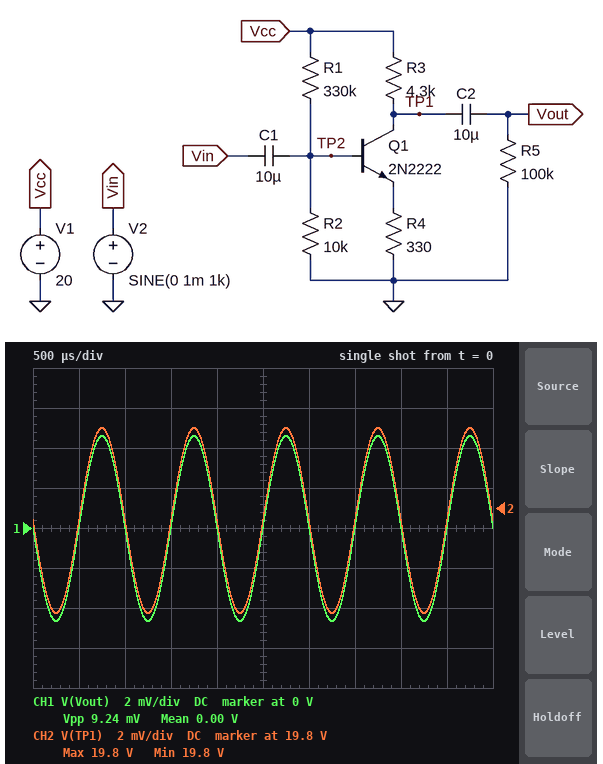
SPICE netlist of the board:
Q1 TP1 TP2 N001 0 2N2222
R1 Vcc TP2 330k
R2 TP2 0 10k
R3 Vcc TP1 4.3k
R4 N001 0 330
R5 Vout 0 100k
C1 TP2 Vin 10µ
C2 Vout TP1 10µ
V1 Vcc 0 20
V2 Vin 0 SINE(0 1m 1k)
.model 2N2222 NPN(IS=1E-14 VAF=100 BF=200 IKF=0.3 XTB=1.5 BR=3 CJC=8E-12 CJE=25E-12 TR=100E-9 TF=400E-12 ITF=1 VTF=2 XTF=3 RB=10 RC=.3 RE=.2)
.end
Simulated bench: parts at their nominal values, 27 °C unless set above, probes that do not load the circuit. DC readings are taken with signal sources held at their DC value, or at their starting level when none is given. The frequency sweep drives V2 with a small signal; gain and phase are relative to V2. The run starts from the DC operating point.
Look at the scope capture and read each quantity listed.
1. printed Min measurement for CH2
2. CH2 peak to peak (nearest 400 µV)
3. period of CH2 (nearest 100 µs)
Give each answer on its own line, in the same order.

19.8 V
9.2 mV
1.0 ms
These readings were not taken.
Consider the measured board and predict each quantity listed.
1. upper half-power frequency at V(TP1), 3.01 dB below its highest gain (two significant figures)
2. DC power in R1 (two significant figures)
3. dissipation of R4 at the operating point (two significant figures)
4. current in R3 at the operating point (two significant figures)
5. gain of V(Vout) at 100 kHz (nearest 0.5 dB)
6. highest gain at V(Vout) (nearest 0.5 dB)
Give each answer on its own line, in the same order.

13 MHz
1.1 mW
710 nW
46 µA
13.5 dB
13.5 dB
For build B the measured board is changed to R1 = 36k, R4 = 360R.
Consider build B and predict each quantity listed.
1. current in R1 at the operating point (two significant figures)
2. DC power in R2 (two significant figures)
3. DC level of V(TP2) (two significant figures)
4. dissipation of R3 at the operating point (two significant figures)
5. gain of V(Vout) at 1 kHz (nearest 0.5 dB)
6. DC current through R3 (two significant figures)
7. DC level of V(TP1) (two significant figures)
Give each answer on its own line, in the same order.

490 µA
540 µW
2.3 V
78 mW
-3.5 dB
4.3 mA
1.7 V
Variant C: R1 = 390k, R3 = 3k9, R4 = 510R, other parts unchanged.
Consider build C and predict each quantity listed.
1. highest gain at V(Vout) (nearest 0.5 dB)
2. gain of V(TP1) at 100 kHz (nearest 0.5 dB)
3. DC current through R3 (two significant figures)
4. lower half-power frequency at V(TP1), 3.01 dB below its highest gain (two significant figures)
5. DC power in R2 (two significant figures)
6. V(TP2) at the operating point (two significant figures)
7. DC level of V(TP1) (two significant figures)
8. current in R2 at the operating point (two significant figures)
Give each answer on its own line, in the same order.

0 dB
-8.5 dB
2.8 µA
9.4 MHz
25 µW
500 mV
20 V
50 µA
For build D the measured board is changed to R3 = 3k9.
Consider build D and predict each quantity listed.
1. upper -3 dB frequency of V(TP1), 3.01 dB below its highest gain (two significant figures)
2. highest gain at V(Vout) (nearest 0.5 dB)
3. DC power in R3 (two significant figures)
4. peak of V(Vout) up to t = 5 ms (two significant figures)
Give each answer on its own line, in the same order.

14 MHz
12.5 dB
8.3 µW
4.2 mV
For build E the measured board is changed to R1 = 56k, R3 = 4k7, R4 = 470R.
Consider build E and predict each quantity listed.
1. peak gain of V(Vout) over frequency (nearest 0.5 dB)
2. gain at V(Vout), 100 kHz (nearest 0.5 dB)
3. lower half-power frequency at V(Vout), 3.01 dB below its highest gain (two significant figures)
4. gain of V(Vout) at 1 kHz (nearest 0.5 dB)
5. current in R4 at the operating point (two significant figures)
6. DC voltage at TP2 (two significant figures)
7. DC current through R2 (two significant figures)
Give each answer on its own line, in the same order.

0 dB
-10.0 dB
570 kHz
-11.5 dB
3.9 mA
2.5 V
250 µA
